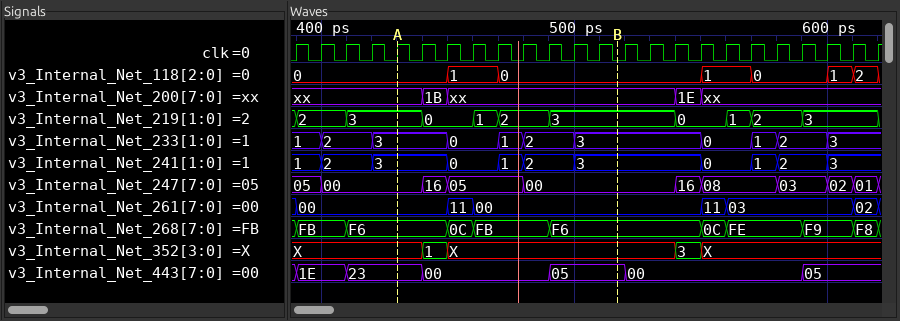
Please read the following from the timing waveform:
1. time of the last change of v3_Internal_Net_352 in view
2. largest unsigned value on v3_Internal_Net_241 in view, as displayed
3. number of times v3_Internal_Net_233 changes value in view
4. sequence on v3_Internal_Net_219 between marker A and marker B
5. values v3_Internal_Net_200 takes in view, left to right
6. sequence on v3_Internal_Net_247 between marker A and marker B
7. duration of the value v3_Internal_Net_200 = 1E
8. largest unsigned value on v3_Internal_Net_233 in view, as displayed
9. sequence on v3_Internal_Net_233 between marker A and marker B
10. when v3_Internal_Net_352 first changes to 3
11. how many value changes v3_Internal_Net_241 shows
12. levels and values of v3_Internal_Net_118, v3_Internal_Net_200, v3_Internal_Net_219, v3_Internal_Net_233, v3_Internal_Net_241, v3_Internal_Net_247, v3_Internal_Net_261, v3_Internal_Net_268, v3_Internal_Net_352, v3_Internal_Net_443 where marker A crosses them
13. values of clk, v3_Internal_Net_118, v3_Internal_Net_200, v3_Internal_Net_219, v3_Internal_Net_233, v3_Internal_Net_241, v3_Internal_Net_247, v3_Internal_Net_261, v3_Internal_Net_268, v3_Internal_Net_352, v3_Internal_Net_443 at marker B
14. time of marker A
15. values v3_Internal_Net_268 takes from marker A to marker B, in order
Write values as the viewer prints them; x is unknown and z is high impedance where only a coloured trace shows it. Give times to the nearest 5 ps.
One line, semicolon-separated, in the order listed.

550 ps; 3; 10; 3, 0, 1, 2, 3; xx, 1B, xx, 1E, xx; 00, 16, 05, 00; 10 ps; 3; 3, 0, 1, 2, 3; 540 ps; 10; v3_Internal_Net_118=0, v3_Internal_Net_200=xx, v3_Internal_Net_219=3, v3_Internal_Net_233=3, v3_Internal_Net_241=3, v3_Internal_Net_247=00, v3_Internal_Net_261=00, v3_Internal_Net_268=F6, v3_Internal_Net_352=X, v3_Internal_Net_443=23; clk=0, v3_Internal_Net_118=0, v3_Internal_Net_200=xx, v3_Internal_Net_219=3, v3_Internal_Net_233=3, v3_Internal_Net_241=3, v3_Internal_Net_247=00, v3_Internal_Net_261=00, v3_Internal_Net_268=F6, v3_Internal_Net_352=X, v3_Internal_Net_443=05; 430 ps; F6, 0C, FB, F6
